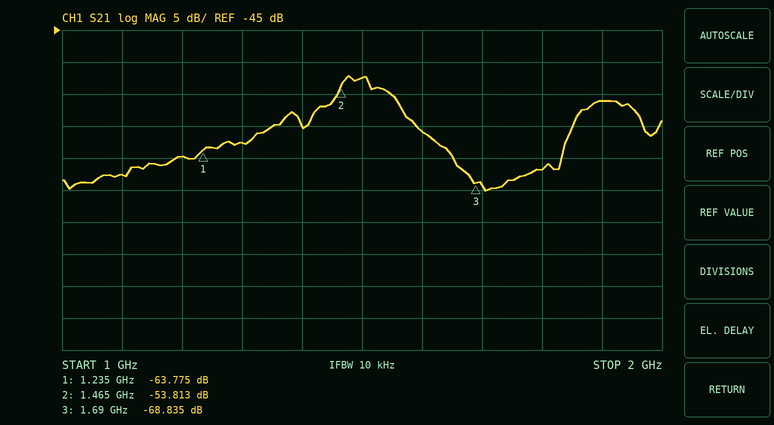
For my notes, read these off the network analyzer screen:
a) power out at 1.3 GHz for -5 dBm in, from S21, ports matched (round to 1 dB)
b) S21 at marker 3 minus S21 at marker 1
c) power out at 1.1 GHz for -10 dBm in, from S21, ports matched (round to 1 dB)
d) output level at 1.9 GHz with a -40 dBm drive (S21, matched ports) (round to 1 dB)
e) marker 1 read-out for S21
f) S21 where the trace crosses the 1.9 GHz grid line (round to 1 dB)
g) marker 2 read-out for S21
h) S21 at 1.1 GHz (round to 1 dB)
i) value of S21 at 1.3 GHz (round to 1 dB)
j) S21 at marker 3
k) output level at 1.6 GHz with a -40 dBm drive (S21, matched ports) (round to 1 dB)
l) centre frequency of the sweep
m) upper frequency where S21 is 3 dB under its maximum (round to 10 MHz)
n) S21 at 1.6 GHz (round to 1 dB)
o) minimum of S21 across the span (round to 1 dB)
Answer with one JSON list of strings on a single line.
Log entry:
["-68 dBm", "-5.060 dB", "-78 dBm", "-96 dBm", "-63.775 dB", "-56 dB", "-53.813 dB", "-68 dB", "-63 dB", "-68.835 dB", "-101 dBm", "1.5 GHz", "1.55 GHz", "-61 dB", "-70 dB"]
